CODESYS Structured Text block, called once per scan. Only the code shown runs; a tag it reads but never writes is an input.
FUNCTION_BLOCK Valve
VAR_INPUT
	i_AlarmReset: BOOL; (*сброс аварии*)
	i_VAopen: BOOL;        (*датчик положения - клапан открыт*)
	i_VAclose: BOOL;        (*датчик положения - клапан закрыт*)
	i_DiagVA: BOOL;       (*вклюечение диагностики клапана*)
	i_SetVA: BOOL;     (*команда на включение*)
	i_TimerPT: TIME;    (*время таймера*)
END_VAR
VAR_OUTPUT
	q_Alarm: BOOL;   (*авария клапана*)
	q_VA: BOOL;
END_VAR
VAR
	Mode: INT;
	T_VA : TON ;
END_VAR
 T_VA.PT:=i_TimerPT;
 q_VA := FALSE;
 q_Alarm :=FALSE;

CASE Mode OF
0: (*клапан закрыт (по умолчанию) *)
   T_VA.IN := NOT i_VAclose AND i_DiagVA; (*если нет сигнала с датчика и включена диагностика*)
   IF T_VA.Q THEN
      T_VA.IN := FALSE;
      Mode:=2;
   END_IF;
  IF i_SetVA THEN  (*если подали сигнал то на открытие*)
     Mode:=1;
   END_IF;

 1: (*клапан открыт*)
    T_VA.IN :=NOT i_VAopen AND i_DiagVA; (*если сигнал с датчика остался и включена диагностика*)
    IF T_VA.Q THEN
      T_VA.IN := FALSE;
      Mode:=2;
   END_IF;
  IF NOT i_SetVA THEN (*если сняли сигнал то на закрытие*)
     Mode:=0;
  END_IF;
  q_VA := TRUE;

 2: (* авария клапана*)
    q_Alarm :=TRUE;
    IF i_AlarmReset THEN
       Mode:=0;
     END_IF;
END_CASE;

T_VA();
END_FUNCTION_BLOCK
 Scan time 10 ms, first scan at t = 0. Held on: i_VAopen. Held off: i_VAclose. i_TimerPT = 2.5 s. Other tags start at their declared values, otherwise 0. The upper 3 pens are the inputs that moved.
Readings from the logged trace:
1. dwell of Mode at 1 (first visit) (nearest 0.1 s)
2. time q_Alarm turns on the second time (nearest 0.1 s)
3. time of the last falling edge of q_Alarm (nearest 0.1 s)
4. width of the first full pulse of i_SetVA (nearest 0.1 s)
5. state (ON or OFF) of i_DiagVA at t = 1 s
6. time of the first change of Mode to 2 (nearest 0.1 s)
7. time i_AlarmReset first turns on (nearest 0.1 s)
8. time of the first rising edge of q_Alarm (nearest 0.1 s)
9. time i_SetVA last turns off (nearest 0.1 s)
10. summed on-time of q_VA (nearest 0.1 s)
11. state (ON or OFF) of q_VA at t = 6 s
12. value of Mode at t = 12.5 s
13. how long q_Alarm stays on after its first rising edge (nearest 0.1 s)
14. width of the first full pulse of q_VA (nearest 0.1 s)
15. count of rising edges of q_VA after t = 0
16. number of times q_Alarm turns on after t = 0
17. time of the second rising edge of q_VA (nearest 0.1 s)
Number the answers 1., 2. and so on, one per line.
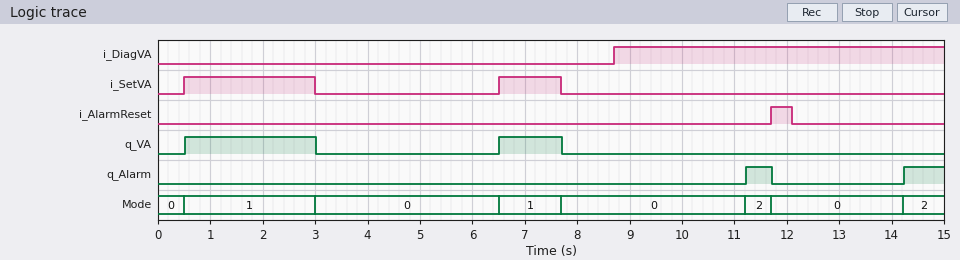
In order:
1. 2.5 s
2. 14.2 s
3. 11.7 s
4. 2.5 s
5. OFF
6. 11.2 s
7. 11.7 s
8. 11.2 s
9. 7.7 s
10. 3.7 s
11. OFF
12. 0
13. 0.5 s
14. 2.5 s
15. 2
16. 2
17. 6.5 s
